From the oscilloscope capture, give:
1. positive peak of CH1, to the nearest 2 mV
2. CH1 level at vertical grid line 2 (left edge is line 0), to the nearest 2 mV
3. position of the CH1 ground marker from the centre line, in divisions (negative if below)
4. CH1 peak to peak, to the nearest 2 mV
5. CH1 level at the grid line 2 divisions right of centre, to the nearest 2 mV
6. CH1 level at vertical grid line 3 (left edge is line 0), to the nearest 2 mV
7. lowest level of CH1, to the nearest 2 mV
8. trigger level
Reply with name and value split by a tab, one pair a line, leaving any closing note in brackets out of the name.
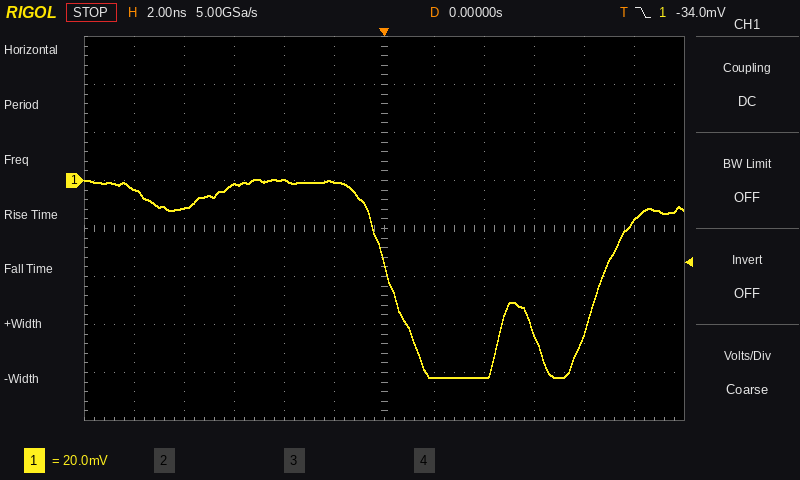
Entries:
positive peak of CH1, to the nearest 2 mV	0 mV
CH1 level at vertical grid line 2 (left edge is line 0), to the nearest 2 mV	-12 mV
position of the CH1 ground marker from the centre line, in divisions	+1.0 div
CH1 peak to peak, to the nearest 2 mV	82 mV
CH1 level at the grid line 2 divisions right of centre, to the nearest 2 mV	-82 mV
CH1 level at vertical grid line 3 (left edge is line 0), to the nearest 2 mV	-2 mV
lowest level of CH1, to the nearest 2 mV	-82 mV
trigger level	-34.0 mV
